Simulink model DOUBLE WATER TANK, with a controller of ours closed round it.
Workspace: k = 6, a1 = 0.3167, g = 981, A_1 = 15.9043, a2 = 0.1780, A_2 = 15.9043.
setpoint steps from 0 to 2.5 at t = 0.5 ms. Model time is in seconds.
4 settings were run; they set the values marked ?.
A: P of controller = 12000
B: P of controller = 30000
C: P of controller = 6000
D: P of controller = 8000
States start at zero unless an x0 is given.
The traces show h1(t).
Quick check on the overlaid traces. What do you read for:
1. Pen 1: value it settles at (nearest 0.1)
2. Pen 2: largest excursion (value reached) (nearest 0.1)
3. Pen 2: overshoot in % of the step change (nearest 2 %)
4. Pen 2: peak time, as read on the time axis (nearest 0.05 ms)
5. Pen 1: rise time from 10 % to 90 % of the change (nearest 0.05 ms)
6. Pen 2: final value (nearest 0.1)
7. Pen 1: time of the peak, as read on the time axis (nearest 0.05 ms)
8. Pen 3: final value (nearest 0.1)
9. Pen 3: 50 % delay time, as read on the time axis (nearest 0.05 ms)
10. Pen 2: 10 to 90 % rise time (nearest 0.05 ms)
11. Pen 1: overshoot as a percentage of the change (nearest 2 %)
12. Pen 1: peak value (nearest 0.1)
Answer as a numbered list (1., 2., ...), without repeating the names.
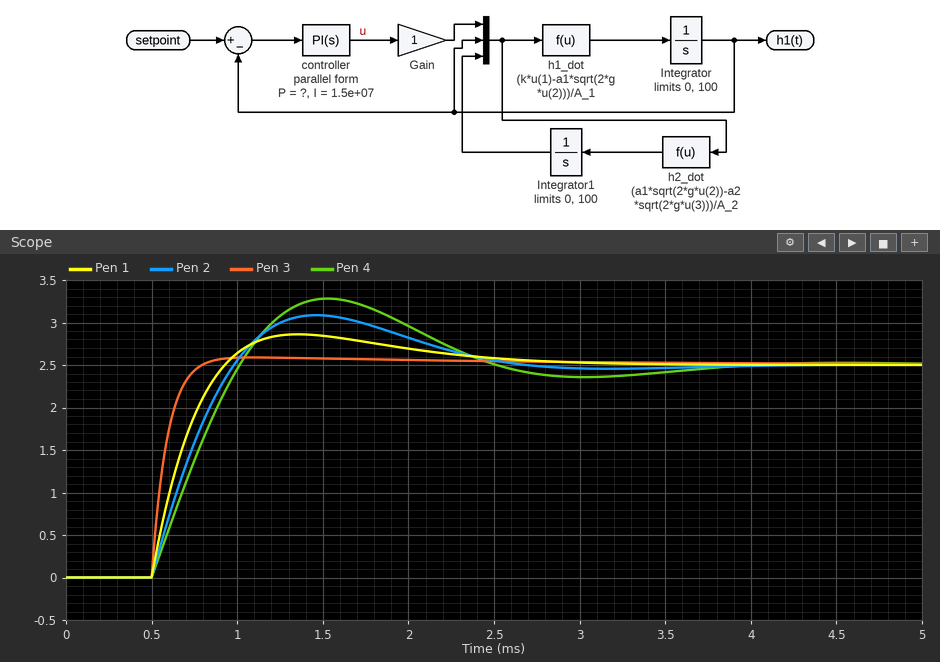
1. 2.5
2. 3.1
3. 24 %
4. 1.45 ms
5. 0.30 ms
6. 2.5
7. 1.35 ms
8. 2.5
9. 0.55 ms
10. 0.35 ms
11. 14 %
12. 2.9
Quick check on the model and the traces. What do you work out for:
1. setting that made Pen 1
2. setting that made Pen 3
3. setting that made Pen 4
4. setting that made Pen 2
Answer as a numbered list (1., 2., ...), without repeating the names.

1. A
2. B
3. C
4. D
